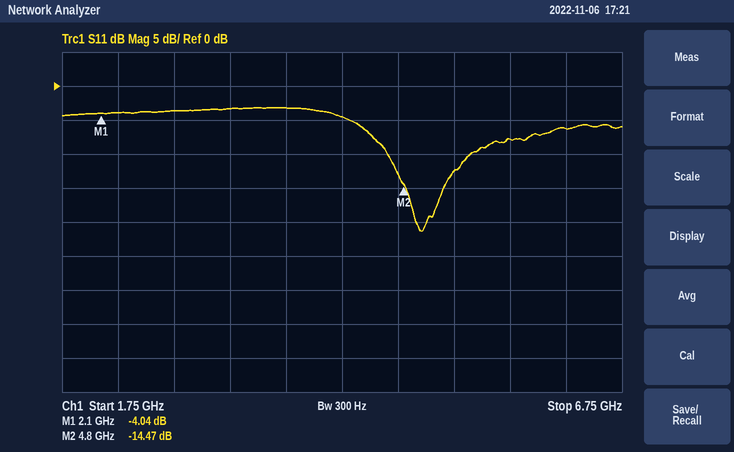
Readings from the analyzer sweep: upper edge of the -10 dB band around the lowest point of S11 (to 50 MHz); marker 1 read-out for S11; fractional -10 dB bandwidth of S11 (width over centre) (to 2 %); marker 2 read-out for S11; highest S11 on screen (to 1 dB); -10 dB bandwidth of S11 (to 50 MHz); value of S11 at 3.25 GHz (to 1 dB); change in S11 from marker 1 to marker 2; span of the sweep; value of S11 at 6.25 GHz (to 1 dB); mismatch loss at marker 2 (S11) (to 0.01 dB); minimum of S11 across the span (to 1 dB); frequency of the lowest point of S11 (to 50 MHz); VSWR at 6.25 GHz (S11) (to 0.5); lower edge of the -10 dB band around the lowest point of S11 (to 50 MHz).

5.40 GHz
-4.04 dB
14 %
-14.47 dB
-3 dB
750 MHz
-3 dB
-10.43 dB
5 GHz
-6 dB
0.16 dB
-21 dB
4.95 GHz
3.0
4.65 GHz
